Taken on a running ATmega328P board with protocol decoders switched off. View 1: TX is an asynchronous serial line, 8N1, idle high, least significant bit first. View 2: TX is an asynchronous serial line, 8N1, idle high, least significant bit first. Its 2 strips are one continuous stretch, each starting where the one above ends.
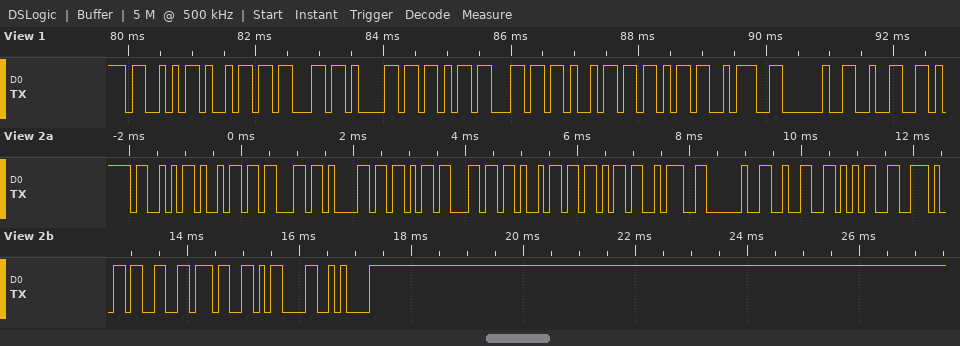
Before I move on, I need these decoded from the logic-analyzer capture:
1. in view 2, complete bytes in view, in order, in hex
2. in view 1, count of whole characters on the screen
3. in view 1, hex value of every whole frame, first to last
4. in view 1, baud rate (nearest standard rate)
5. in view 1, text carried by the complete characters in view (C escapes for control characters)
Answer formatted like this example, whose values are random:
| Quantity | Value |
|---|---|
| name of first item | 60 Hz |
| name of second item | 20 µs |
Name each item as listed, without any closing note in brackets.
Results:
| Quantity | Value |
|---|---|
| in view 2, complete bytes in view, in order, in hex | 53 69 63 61 6B 6C 69 6B 3A 20 32 35 2E 33 37 0D 0A |
| in view 1, count of whole characters on the screen | 11 |
| in view 1, hex value of every whole frame, first to last | 53 69 63 61 6B 6C 69 6B 3A 20 32 |
| in view 1, baud rate | 9600 baud |
| in view 1, text carried by the complete characters in view | "Sicaklik: 2" |
